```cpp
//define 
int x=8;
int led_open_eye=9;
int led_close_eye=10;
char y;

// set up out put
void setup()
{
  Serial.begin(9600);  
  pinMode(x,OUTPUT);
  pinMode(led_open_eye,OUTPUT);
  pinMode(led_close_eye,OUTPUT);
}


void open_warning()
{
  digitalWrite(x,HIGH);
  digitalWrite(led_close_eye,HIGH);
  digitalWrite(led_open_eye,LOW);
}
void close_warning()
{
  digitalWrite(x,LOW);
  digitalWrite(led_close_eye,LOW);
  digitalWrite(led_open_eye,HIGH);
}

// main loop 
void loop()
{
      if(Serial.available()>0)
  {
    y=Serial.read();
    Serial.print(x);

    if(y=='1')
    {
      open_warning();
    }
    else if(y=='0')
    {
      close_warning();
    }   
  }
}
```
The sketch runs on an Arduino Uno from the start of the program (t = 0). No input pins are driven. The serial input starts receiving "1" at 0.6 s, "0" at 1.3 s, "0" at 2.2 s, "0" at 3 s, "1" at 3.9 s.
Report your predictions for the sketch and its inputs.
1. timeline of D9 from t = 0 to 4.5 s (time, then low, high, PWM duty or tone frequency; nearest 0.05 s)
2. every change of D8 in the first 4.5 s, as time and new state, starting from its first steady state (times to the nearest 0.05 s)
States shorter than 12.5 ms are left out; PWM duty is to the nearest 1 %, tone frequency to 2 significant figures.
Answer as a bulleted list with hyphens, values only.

- 0 s low; 1.3 s high; 3.9 s low
- 0 s low; 0.6 s high; 1.3 s low; 3.9 s high
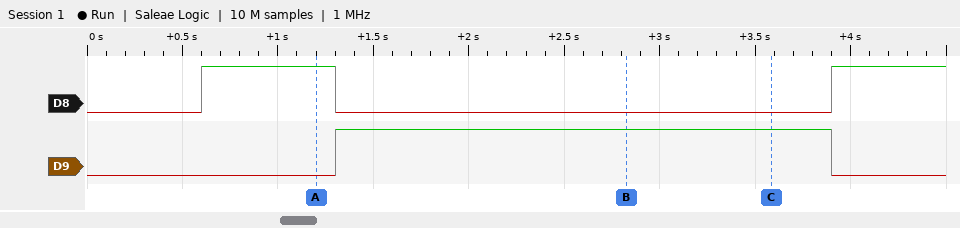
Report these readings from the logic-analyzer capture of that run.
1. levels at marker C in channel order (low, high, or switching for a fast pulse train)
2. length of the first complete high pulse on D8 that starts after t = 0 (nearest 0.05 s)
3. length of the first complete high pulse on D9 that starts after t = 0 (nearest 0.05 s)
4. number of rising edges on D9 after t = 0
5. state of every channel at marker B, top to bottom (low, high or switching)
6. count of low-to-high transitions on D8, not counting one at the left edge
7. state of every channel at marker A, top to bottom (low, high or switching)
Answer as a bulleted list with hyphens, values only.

- D8 low, D9 high
- 0.70 s
- 2.60 s
- 1
- D8 low, D9 high
- 2
- D8 high, D9 low
